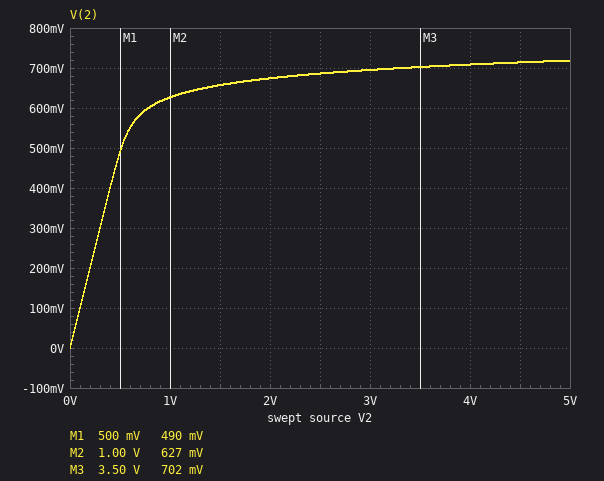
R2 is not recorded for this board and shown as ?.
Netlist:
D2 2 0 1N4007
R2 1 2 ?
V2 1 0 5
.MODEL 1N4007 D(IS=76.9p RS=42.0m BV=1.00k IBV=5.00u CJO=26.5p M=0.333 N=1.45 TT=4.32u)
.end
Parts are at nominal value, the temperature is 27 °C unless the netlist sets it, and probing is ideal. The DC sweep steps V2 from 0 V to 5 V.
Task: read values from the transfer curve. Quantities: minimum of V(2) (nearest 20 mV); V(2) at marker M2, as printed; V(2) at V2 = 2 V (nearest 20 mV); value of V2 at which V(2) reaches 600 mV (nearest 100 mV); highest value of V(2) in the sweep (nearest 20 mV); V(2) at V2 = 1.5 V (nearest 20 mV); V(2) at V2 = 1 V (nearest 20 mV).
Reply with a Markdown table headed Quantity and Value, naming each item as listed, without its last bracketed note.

| Quantity | Value |
|---|---|
| minimum of V(2) | 0 V |
| V(2) at marker M2, as printed | 627 mV |
| V(2) at V2 = 2 V | 680 mV |
| value of V2 at which V(2) reaches 600 mV | 800 mV |
| highest value of V(2) in the sweep | 720 mV |
| V(2) at V2 = 1.5 V | 660 mV |
| V(2) at V2 = 1 V | 620 mV |
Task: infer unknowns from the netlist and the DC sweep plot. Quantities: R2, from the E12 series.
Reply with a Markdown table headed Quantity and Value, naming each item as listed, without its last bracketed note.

| Quantity | Value |
|---|---|
| R2, from the E12 series | 270 Ω |
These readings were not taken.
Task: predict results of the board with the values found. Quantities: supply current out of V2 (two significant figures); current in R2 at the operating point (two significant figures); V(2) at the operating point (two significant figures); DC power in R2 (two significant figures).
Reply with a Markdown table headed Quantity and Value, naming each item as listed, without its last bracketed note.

| Quantity | Value |
|---|---|
| supply current out of V2 | 16 mA |
| current in R2 at the operating point | 16 mA |
| V(2) at the operating point | 720 mV |
| DC power in R2 | 68 mW |
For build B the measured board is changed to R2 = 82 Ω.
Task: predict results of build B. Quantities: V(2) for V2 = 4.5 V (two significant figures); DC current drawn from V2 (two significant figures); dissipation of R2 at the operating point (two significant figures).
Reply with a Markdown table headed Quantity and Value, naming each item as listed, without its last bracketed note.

| Quantity | Value |
|---|---|
| V(2) for V2 = 4.5 V | 760 mV |
| DC current drawn from V2 | 52 mA |
| dissipation of R2 at the operating point | 220 mW |
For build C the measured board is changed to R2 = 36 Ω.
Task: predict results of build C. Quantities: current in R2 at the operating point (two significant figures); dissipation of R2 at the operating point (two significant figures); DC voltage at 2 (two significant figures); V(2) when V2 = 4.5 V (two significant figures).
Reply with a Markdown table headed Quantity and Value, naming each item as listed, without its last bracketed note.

| Quantity | Value |
|---|---|
| current in R2 at the operating point | 120 mA |
| dissipation of R2 at the operating point | 490 mW |
| DC voltage at 2 | 800 mV |
| V(2) when V2 = 4.5 V | 790 mV |
